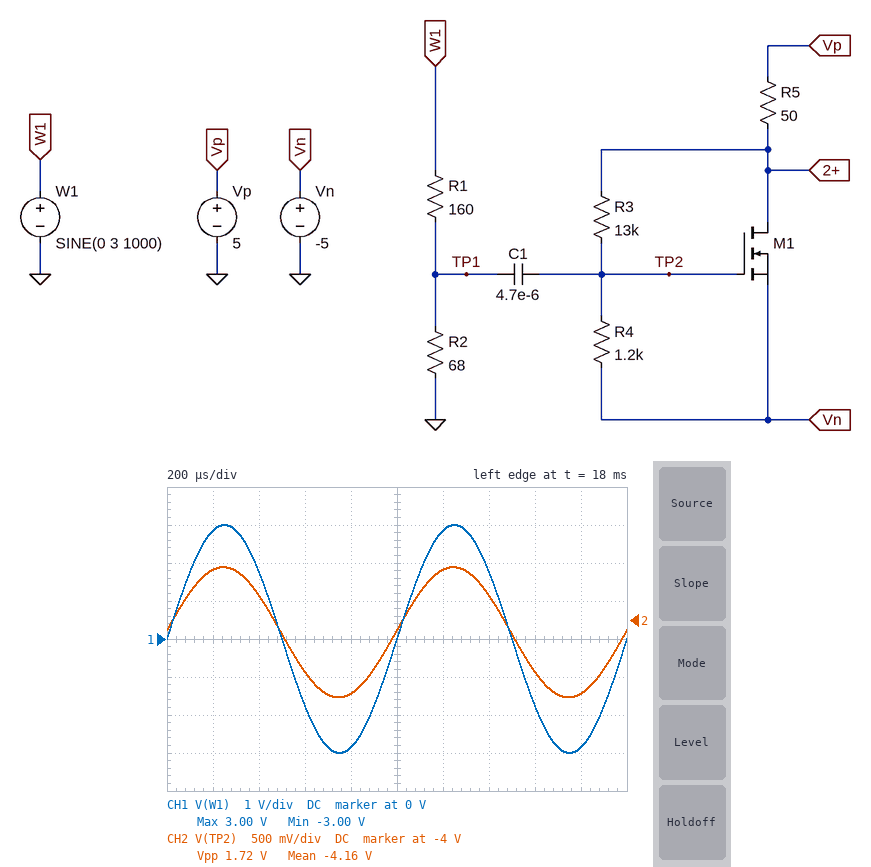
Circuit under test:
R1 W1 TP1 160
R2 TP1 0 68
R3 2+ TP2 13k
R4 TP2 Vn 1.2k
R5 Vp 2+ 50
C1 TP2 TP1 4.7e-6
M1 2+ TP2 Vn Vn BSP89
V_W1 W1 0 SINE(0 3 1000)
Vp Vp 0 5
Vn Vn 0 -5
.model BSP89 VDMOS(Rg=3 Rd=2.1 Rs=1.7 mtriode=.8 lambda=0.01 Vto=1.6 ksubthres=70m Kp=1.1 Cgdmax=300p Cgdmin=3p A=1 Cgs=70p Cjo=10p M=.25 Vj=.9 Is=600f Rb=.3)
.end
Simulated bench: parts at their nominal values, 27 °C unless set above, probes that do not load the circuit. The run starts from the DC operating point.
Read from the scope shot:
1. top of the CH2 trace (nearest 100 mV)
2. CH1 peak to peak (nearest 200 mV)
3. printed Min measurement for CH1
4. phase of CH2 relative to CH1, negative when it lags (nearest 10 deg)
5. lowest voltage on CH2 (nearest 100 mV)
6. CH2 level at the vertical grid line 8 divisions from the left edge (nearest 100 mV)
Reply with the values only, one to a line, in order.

-3.3 V
6.0 V
-3.00 V
0 deg
-5.0 V
-4.7 V
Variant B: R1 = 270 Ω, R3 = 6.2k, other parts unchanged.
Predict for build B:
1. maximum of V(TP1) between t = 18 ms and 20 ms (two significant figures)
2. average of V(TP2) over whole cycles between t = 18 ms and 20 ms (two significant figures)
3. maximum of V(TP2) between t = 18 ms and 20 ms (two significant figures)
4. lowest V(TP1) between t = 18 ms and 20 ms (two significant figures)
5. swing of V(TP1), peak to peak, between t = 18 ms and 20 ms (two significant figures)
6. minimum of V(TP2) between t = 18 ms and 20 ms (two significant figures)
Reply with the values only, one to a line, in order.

550 mV
-3.5 V
-3.0 V
-570 mV
1.1 V
-4.1 V
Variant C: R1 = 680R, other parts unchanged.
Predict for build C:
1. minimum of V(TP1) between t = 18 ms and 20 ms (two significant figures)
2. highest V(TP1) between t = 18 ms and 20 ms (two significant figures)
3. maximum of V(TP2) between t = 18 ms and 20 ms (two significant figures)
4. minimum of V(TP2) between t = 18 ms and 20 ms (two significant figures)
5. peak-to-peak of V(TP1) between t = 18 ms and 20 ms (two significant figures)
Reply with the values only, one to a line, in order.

-260 mV
260 mV
-3.9 V
-4.4 V
520 mV
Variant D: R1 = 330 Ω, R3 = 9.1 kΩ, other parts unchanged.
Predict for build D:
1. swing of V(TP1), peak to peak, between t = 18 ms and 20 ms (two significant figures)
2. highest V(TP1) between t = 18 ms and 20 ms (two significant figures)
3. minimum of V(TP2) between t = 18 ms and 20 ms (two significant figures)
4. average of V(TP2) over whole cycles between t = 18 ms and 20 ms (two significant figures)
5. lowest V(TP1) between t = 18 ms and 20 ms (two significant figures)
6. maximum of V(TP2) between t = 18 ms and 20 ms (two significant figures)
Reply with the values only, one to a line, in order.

970 mV
490 mV
-4.3 V
-3.8 V
-490 mV
-3.4 V
